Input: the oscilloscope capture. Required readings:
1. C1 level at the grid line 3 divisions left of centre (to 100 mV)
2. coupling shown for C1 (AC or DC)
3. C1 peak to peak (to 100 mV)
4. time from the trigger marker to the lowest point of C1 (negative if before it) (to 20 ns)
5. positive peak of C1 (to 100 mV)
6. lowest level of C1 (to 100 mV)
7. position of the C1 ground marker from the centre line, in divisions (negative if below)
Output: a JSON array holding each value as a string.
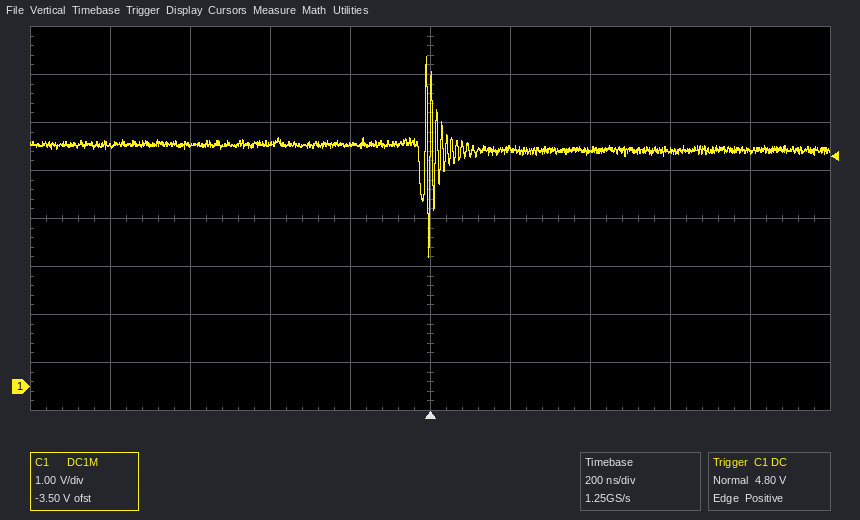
["5.0 V", "DC", "4.2 V", "0 ns", "6.9 V", "2.7 V", "-3.5 div"]
